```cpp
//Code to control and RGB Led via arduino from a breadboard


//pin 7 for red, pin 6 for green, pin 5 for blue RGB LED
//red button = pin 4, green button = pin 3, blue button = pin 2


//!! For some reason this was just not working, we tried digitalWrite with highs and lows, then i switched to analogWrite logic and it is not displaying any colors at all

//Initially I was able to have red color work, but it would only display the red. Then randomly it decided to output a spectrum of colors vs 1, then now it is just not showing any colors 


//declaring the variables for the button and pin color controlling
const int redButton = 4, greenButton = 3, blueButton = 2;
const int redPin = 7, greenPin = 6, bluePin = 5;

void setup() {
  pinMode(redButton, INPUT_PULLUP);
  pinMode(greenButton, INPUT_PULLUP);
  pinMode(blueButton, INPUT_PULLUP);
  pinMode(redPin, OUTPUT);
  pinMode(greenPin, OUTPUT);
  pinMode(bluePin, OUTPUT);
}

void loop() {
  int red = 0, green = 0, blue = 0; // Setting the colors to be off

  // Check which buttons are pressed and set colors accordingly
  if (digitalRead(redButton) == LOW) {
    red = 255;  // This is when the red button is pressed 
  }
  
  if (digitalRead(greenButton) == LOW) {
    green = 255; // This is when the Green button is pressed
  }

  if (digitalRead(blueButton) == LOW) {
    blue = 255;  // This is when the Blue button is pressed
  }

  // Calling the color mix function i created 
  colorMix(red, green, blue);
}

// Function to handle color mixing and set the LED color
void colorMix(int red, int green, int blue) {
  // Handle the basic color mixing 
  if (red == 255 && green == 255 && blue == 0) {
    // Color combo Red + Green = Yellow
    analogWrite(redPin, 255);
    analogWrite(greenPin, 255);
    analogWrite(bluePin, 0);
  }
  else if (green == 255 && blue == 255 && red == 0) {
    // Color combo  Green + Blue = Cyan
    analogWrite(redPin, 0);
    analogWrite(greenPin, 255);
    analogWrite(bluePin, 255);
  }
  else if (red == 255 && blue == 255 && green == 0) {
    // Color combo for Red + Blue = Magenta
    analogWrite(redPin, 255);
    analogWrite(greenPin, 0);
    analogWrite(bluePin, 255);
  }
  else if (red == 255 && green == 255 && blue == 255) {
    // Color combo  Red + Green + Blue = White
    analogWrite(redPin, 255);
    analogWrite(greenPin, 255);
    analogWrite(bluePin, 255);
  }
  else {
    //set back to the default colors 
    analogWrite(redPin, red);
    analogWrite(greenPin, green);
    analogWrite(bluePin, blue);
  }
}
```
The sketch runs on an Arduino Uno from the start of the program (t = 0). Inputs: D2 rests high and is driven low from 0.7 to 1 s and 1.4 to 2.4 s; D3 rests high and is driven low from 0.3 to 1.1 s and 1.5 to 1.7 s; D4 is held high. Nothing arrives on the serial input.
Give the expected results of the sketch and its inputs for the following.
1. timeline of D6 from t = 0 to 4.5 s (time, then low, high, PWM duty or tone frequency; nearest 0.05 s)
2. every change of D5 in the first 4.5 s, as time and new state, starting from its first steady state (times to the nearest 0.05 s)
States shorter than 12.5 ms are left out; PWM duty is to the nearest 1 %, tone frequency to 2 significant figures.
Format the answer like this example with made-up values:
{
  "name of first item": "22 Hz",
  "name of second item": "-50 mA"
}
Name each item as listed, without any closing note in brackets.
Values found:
{
  "timeline of D6 from t = 0 to 4.5 s": "0 s low; 0.3 s high; 1.1 s low; 1.5 s high; 1.7 s low",
  "every change of D5 in the first 4.5 s, as time and new state, starting from its first steady state": "0 s low; 0.7 s high; 1 s low; 1.4 s high; 2.4 s low"
}
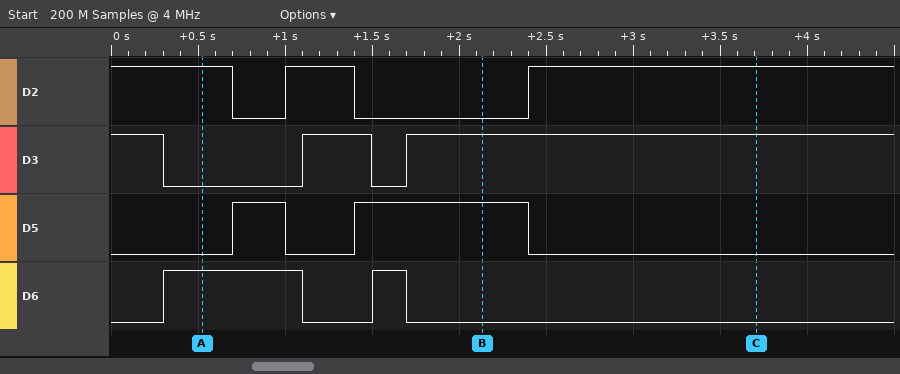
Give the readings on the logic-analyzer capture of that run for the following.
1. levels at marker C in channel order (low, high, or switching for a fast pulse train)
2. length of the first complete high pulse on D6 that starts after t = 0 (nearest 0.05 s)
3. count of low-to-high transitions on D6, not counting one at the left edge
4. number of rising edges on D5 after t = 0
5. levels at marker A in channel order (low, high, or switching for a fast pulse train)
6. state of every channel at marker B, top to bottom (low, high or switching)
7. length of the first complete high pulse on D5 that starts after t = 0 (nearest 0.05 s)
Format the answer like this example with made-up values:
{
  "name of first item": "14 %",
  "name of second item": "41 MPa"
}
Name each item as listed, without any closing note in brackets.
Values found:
{
  "levels at marker C in channel order": "D2 high, D3 high, D5 low, D6 low",
  "length of the first complete high pulse on D6 that starts after t = 0": "0.80 s",
  "count of low-to-high transitions on D6, not counting one at the left edge": "2",
  "number of rising edges on D5 after t = 0": "2",
  "levels at marker A in channel order": "D2 high, D3 low, D5 low, D6 high",
  "state of every channel at marker B, top to bottom": "D2 low, D3 high, D5 high, D6 low",
  "length of the first complete high pulse on D5 that starts after t = 0": "0.30 s"
}
